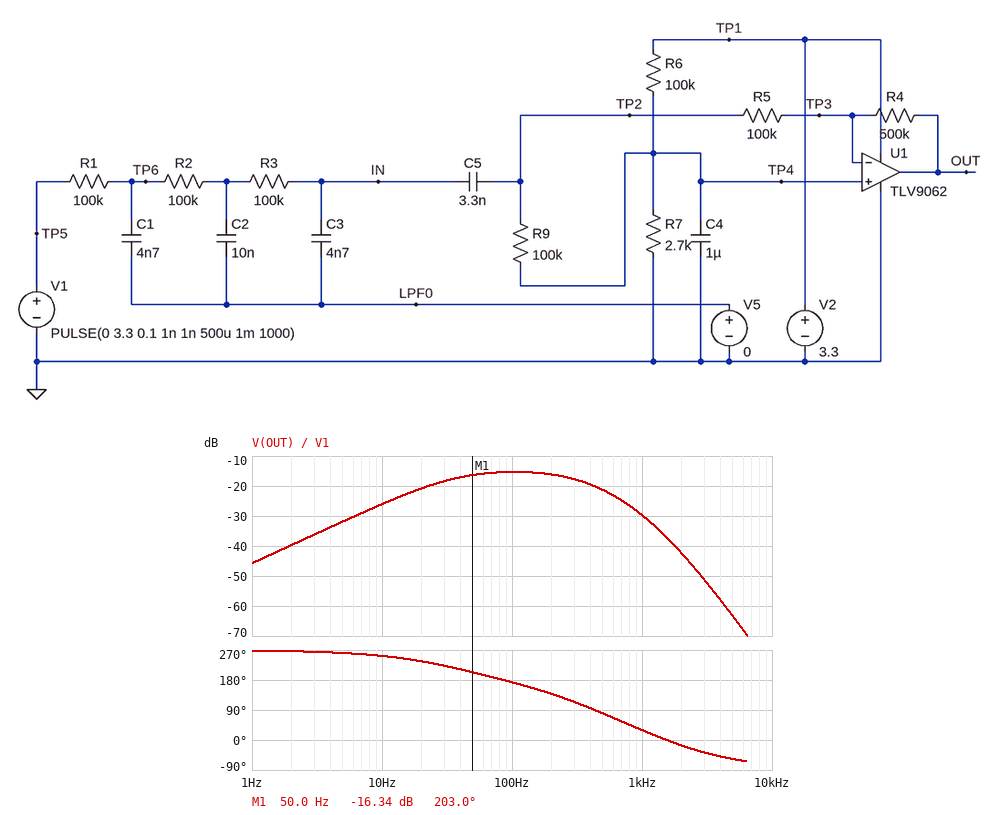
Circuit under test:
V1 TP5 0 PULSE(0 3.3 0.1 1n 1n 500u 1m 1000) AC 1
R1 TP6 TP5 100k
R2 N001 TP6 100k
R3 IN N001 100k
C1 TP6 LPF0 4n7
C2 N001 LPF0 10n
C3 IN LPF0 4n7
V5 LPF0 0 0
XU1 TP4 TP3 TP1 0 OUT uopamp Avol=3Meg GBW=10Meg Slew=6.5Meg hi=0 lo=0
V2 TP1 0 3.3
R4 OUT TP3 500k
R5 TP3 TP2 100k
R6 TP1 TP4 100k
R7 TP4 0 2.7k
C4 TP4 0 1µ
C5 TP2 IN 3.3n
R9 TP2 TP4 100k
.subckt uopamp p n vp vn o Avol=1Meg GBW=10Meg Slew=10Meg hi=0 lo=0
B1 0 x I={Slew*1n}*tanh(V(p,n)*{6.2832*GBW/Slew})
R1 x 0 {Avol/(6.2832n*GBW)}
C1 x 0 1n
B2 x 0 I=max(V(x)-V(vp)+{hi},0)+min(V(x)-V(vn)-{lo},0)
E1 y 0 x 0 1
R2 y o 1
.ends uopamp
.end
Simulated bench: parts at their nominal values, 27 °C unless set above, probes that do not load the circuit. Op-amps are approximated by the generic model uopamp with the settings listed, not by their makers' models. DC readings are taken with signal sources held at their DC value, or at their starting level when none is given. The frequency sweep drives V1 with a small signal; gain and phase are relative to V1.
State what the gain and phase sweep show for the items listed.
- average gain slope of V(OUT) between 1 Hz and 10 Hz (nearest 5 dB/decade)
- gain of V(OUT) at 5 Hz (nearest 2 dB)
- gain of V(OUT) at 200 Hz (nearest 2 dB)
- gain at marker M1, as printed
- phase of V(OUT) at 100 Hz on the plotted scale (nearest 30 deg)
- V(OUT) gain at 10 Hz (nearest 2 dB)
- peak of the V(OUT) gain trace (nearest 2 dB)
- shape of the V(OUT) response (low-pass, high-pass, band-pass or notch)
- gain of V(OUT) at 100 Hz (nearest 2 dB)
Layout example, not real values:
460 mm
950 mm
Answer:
20 dB/decade
-32 dB
-16 dB
-16.34 dB
180 deg
-26 dB
-16 dB
band-pass
-16 dB
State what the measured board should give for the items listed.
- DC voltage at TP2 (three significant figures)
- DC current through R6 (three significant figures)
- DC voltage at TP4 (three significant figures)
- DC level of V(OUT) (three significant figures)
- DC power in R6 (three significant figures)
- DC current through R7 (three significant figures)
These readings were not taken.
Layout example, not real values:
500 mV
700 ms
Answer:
86.8 mV
32.1 µA
86.8 mV
86.8 mV
103 µW
32.1 µA
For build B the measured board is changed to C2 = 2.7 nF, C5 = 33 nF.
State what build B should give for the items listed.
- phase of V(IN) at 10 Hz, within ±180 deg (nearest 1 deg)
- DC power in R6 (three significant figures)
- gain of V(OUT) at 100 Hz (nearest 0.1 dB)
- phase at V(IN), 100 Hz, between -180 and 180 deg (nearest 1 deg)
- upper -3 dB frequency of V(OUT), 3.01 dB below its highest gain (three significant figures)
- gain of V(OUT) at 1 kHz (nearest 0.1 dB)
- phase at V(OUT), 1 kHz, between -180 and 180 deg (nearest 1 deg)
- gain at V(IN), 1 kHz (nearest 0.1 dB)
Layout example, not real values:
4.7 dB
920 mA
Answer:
-36 deg
103 µW
-4.6 dB
-63 deg
324 Hz
-18.4 dB
32 deg
-32.4 dB
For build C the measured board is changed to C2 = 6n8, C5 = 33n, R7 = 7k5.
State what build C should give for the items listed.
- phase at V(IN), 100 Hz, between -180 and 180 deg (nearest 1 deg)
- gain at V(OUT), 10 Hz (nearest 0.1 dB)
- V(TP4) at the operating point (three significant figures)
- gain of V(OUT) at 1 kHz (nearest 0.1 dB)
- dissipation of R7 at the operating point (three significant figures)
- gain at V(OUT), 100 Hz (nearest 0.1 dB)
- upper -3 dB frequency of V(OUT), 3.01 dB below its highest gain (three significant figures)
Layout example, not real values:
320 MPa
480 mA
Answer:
-73 deg
-8.3 dB
230 mV
-23.8 dB
7.07 µW
-5.4 dB
229 Hz
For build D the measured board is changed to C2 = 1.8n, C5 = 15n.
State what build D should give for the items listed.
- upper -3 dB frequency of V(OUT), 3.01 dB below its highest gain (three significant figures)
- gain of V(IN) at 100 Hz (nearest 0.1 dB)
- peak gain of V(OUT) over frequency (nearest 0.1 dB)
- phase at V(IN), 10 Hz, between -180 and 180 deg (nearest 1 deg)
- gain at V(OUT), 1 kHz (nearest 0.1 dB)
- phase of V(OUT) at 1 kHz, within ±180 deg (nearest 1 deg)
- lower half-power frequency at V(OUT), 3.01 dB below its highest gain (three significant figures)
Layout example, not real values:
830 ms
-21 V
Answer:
392 Hz
-12.3 dB
-5.8 dB
-23 deg
-17.4 dB
45 deg
20.8 Hz
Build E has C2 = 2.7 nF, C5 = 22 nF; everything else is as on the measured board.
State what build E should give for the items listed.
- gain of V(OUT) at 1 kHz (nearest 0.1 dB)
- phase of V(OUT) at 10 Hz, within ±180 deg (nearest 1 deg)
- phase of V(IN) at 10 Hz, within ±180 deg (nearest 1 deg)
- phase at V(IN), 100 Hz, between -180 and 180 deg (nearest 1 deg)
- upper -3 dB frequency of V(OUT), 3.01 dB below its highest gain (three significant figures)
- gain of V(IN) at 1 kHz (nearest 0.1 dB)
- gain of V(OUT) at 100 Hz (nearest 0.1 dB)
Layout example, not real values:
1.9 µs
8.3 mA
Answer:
-18.6 dB
-123 deg
-29 deg
-71 deg
341 Hz
-32.5 dB
-5.2 dB
